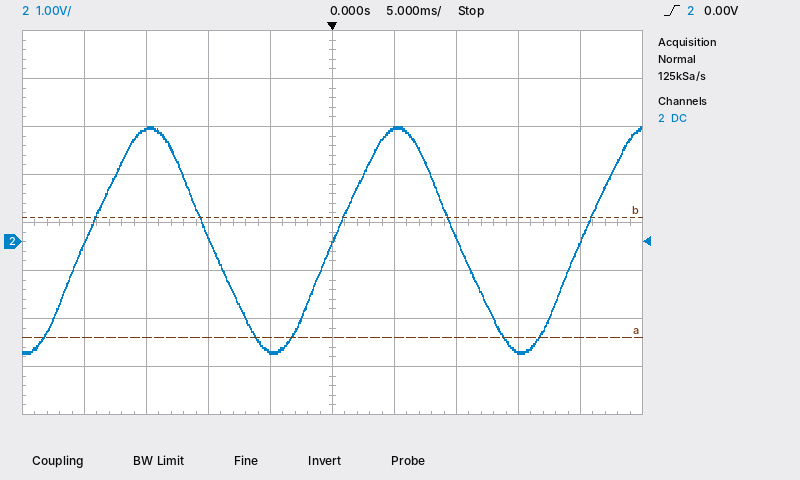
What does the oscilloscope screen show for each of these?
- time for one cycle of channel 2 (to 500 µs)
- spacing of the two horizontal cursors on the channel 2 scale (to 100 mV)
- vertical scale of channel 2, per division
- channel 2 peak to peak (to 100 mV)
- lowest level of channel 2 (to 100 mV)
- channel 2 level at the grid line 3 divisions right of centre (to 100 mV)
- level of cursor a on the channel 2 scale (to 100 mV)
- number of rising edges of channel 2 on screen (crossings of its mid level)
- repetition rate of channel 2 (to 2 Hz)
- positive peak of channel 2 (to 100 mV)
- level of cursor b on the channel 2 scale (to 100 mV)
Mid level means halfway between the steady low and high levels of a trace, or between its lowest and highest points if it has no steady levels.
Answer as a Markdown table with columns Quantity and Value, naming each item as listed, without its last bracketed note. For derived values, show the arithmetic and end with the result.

| Quantity | Value |
|---|---|
| time for one cycle of channel 2 | 20.0 ms |
| spacing of the two horizontal cursors on the channel 2 scale | 2.5 V |
| vertical scale of channel 2, per division | 1 V |
| channel 2 peak to peak | 2.4 V − (-2.3 V) = 4.7 V |
| lowest level of channel 2 | -2.3 V |
| channel 2 level at the grid line 3 divisions right of centre | -2.3 V |
| level of cursor a on the channel 2 scale | -2.0 V |
| number of rising edges of channel 2 on screen | 3 |
| repetition rate of channel 2 | 1 / 20.0 ms ≈ 50 Hz |
| positive peak of channel 2 | 2.4 V |
| level of cursor b on the channel 2 scale | 500 mV |
